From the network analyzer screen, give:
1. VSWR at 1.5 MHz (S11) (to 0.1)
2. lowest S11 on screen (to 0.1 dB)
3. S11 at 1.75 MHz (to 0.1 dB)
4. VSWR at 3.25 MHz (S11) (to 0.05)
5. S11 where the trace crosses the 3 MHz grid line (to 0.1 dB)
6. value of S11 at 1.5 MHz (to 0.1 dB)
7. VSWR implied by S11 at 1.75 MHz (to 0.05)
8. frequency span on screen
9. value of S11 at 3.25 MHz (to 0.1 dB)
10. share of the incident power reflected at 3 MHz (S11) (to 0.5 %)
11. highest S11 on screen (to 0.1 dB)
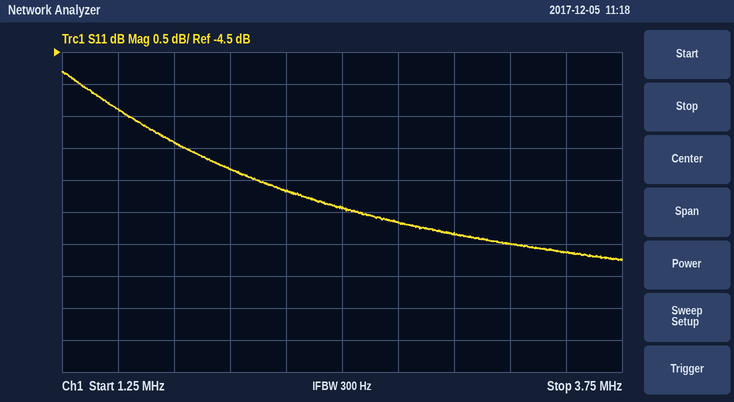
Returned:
3.3
-7.8 dB
-5.9 dB
2.45
-7.3 dB
-5.4 dB
3.05
2.5 MHz
-7.5 dB
18.5 %
-4.8 dB
